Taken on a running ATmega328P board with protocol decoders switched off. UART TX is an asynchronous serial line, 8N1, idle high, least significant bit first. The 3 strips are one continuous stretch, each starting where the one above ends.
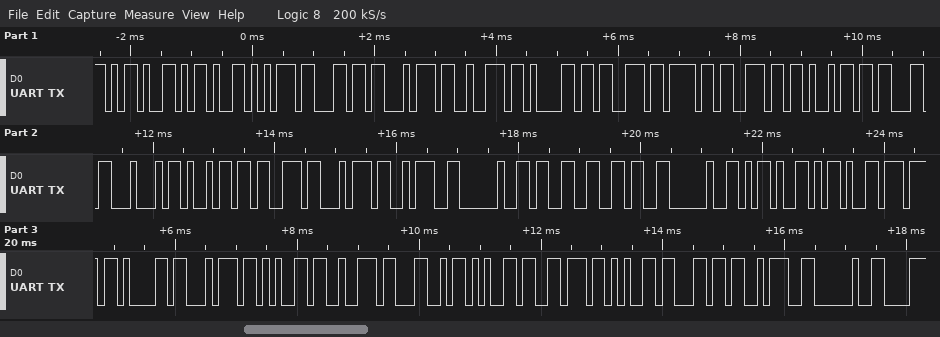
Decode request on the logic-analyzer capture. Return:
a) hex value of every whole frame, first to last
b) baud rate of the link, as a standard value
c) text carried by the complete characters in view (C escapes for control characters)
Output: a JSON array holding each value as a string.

["0x2D 0x2D 0x75 0x6C 0x74 0x72 0x61 0x73 0x6F 0x6E 0x69 0x63 0x44 0x69 0x73 0x74 0x3A 0x20 0x33 0x36 0x20 0x2D 0x2D 0x77 0x61 0x74 0x65 0x72 0x4C 0x65 0x76 0x65 0x6C 0x3A 0x20", "9600 baud", "\"--ultrasonicDist: 36 --waterLevel: \""]
